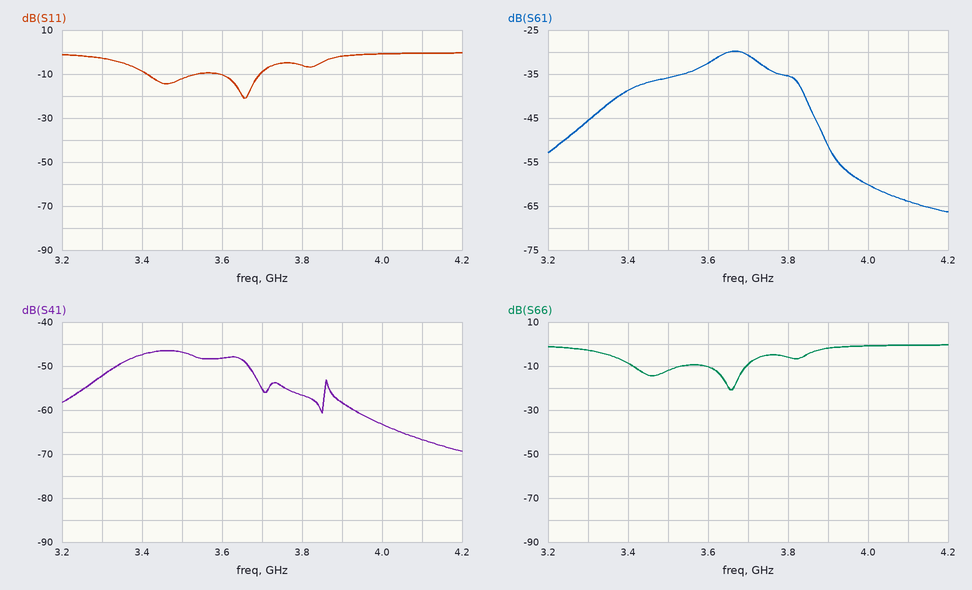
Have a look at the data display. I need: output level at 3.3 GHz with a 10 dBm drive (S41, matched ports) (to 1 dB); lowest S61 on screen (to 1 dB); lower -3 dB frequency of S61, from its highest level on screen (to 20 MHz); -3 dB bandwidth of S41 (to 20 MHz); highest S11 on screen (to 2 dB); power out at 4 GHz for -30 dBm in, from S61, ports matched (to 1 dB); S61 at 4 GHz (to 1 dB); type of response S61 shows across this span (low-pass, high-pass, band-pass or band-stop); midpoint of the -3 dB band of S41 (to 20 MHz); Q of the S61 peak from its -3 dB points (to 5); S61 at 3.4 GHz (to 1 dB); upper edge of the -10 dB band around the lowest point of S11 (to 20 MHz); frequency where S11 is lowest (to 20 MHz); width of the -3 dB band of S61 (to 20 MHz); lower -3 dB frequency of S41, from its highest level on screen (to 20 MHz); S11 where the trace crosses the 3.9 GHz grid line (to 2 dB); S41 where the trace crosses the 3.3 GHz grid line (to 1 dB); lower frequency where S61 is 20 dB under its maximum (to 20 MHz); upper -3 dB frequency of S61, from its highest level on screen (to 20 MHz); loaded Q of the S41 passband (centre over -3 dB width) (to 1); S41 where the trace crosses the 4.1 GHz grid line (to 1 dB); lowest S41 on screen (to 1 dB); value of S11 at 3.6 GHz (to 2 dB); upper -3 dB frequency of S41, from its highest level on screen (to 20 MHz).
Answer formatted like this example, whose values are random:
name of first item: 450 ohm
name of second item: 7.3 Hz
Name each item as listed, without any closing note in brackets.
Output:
output level at 3.3 GHz with a 10 dBm drive (S41, matched ports): -42 dBm
lowest S61 on screen: -66 dB
lower -3 dB frequency of S61, from its highest level on screen: 3.60 GHz
-3 dB bandwidth of S41: 320 MHz
highest S11 on screen: 0 dB
power out at 4 GHz for -30 dBm in, from S61, ports matched: -90 dBm
S61 at 4 GHz: -60 dB
type of response S61 shows across this span: band-pass
midpoint of the -3 dB band of S41: 3.50 GHz
Q of the S61 peak from its -3 dB points: 25
S61 at 3.4 GHz: -39 dB
upper edge of the -10 dB band around the lowest point of S11: 3.70 GHz
frequency where S11 is lowest: 3.66 GHz
width of the -3 dB band of S61: 140 MHz
lower -3 dB frequency of S41, from its highest level on screen: 3.34 GHz
S11 where the trace crosses the 3.9 GHz grid line: -2 dB
S41 where the trace crosses the 3.3 GHz grid line: -52 dB
lower frequency where S61 is 20 dB under its maximum: 3.24 GHz
upper -3 dB frequency of S61, from its highest level on screen: 3.74 GHz
loaded Q of the S41 passband (centre over -3 dB width): 11
S41 where the trace crosses the 4.1 GHz grid line: -67 dB
lowest S41 on screen: -69 dB
value of S11 at 3.6 GHz: -10 dB
upper -3 dB frequency of S41, from its highest level on screen: 3.66 GHz
